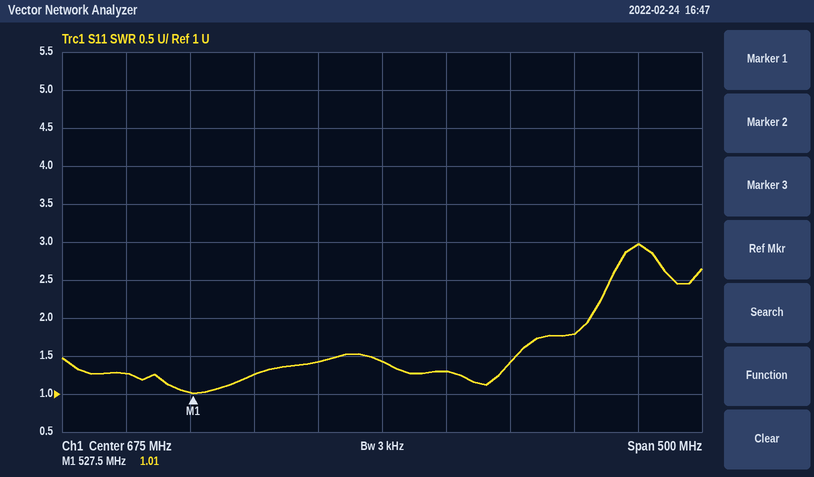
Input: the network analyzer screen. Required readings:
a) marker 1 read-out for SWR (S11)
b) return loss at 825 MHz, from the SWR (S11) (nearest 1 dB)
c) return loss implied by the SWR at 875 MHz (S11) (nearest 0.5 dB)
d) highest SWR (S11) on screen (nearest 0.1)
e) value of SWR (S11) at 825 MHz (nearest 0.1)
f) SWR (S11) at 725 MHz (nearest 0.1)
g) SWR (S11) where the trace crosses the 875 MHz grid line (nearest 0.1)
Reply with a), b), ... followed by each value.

a) 1.01
b) 11 dB
c) 6.0 dB
d) 3.0
e) 1.8
f) 1.3
g) 3.0
